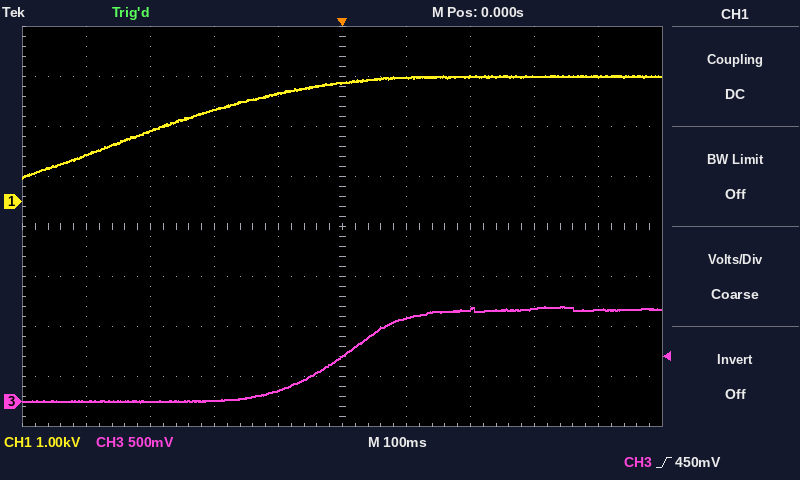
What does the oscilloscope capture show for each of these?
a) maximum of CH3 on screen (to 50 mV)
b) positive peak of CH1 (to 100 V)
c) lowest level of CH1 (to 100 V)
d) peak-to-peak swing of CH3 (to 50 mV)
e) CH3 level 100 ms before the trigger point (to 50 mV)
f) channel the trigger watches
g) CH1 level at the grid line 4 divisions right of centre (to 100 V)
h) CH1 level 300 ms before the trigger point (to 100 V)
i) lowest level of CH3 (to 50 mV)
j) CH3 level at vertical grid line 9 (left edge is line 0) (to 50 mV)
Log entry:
950 mV
2.5 kV
500 V
950 mV
100 mV
CH3
2.5 kV
1.4 kV
0 mV
900 mV
